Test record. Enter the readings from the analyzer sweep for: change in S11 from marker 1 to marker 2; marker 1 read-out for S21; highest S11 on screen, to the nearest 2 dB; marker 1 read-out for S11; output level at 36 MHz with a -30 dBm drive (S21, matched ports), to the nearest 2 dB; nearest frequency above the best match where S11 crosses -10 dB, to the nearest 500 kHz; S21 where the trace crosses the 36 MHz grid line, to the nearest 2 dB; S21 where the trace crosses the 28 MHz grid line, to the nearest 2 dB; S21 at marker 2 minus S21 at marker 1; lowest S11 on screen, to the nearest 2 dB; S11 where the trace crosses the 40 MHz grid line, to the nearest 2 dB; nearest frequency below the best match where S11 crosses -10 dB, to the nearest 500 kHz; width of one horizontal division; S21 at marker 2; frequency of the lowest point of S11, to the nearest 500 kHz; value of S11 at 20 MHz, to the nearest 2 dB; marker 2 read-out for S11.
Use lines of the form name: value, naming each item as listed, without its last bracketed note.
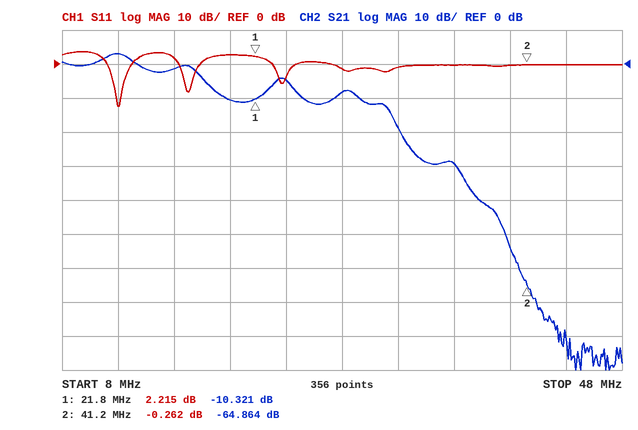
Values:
change in S11 from marker 1 to marker 2: -2.477 dB
marker 1 read-out for S21: -10.321 dB
highest S11 on screen, to the nearest 2 dB: 4 dB
marker 1 read-out for S11: 2.215 dB
output level at 36 MHz with a -30 dBm drive (S21, matched ports), to the nearest 2 dB: -60 dBm
nearest frequency above the best match where S11 crosses -10 dB, to the nearest 500 kHz: 12.0 MHz
S21 where the trace crosses the 36 MHz grid line, to the nearest 2 dB: -30 dB
S21 where the trace crosses the 28 MHz grid line, to the nearest 2 dB: -8 dB
S21 at marker 2 minus S21 at marker 1: -54.543 dB
lowest S11 on screen, to the nearest 2 dB: -12 dB
S11 where the trace crosses the 40 MHz grid line, to the nearest 2 dB: 0 dB
nearest frequency below the best match where S11 crosses -10 dB, to the nearest 500 kHz: 12.0 MHz
width of one horizontal division: 4 MHz
S21 at marker 2: -64.864 dB
frequency of the lowest point of S11, to the nearest 500 kHz: 12.0 MHz
value of S11 at 20 MHz, to the nearest 2 dB: 2 dB
marker 2 read-out for S11: -0.262 dB
